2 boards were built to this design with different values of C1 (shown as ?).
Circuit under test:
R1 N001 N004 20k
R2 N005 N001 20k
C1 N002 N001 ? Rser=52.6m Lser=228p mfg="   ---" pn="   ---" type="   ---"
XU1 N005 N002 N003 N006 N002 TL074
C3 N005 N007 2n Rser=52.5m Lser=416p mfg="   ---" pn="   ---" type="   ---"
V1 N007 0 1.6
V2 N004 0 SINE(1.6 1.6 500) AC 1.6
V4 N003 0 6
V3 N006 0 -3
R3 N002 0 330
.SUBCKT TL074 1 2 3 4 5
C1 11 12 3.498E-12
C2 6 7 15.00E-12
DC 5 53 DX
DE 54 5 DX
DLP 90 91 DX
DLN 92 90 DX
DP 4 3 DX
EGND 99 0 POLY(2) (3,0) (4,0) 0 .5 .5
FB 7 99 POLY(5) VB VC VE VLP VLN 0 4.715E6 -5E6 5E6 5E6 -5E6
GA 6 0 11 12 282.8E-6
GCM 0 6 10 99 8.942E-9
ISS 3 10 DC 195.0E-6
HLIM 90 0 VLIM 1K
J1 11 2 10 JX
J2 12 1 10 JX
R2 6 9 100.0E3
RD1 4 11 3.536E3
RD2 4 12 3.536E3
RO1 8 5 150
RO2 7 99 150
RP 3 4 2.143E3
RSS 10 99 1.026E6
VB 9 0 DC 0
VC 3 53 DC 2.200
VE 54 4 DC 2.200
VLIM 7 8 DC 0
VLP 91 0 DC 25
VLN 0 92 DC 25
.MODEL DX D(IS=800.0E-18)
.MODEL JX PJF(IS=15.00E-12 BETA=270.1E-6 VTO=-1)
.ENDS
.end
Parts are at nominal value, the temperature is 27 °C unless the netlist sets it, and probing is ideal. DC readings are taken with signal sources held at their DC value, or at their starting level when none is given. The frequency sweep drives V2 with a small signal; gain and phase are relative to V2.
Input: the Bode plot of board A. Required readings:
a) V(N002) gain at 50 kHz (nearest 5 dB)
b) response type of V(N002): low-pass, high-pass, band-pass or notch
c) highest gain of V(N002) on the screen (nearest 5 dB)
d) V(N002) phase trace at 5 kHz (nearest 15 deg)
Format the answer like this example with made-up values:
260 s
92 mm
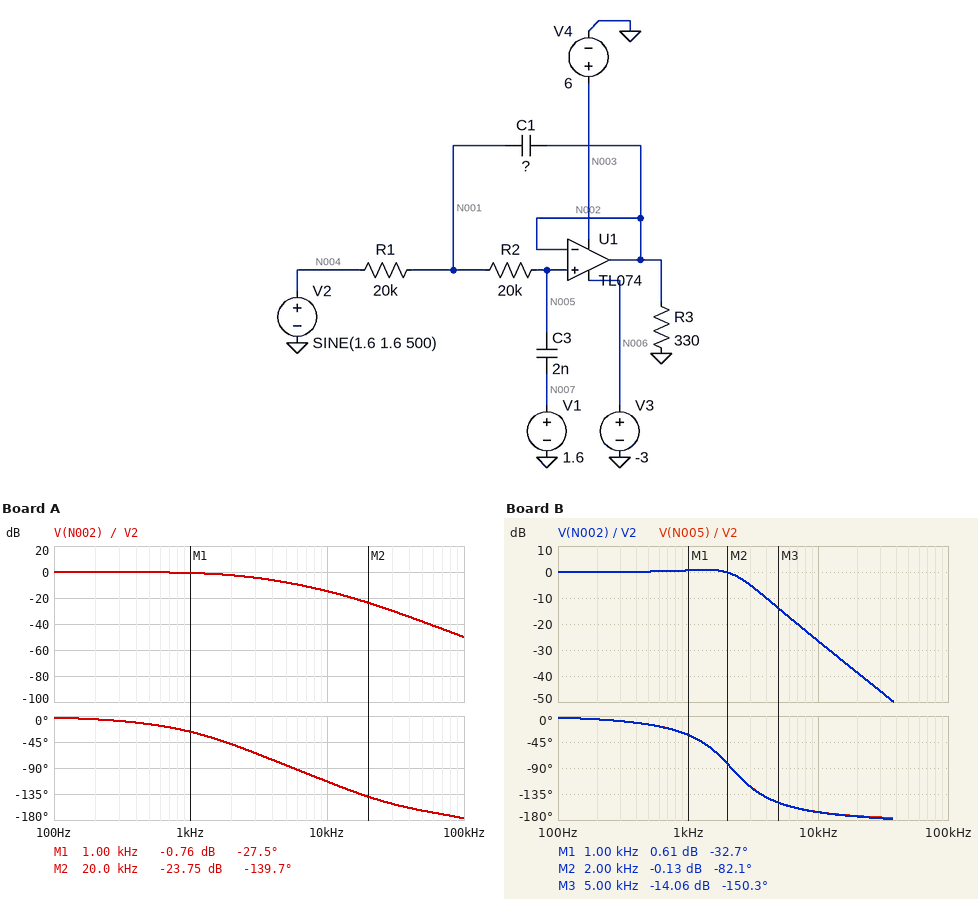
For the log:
-40 dB
low-pass
0 dB
-90 deg
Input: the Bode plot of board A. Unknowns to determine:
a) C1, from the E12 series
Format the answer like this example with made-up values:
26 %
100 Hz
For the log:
1 nF
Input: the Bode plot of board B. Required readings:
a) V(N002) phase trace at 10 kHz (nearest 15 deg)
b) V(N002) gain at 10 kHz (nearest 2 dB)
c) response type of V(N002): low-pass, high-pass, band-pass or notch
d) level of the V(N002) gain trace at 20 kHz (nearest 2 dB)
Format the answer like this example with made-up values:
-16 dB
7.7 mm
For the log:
-165 deg
-26 dB
low-pass
-38 dB
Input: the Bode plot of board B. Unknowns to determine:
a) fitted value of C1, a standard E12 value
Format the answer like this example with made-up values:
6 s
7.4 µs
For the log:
6.8 nF
